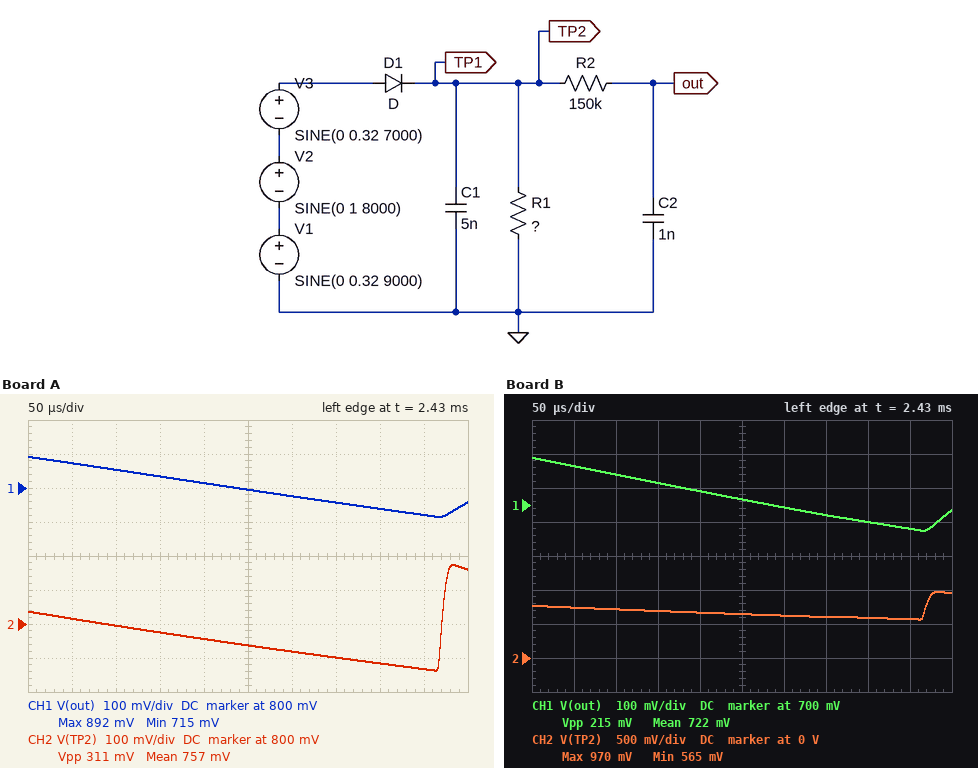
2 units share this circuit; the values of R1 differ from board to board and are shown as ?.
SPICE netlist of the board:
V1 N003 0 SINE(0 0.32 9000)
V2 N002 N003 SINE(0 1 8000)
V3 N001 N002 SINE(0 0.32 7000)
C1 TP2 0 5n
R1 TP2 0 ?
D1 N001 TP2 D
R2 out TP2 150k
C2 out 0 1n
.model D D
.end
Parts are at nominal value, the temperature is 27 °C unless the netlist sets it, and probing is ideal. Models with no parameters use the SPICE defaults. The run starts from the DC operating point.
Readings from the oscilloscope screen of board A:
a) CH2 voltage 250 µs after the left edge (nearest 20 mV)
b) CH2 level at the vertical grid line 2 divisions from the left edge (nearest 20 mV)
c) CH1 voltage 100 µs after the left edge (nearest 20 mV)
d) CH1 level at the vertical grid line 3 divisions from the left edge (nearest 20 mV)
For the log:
740 mV
800 mV
860 mV
840 mV
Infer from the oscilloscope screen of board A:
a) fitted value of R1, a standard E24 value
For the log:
330 kΩ
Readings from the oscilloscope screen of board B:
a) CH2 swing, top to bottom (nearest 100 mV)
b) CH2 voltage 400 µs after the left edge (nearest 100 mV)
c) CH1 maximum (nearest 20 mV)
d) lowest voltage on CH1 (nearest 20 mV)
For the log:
400 mV
600 mV
840 mV
620 mV
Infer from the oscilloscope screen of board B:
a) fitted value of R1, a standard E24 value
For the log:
240 kΩ
